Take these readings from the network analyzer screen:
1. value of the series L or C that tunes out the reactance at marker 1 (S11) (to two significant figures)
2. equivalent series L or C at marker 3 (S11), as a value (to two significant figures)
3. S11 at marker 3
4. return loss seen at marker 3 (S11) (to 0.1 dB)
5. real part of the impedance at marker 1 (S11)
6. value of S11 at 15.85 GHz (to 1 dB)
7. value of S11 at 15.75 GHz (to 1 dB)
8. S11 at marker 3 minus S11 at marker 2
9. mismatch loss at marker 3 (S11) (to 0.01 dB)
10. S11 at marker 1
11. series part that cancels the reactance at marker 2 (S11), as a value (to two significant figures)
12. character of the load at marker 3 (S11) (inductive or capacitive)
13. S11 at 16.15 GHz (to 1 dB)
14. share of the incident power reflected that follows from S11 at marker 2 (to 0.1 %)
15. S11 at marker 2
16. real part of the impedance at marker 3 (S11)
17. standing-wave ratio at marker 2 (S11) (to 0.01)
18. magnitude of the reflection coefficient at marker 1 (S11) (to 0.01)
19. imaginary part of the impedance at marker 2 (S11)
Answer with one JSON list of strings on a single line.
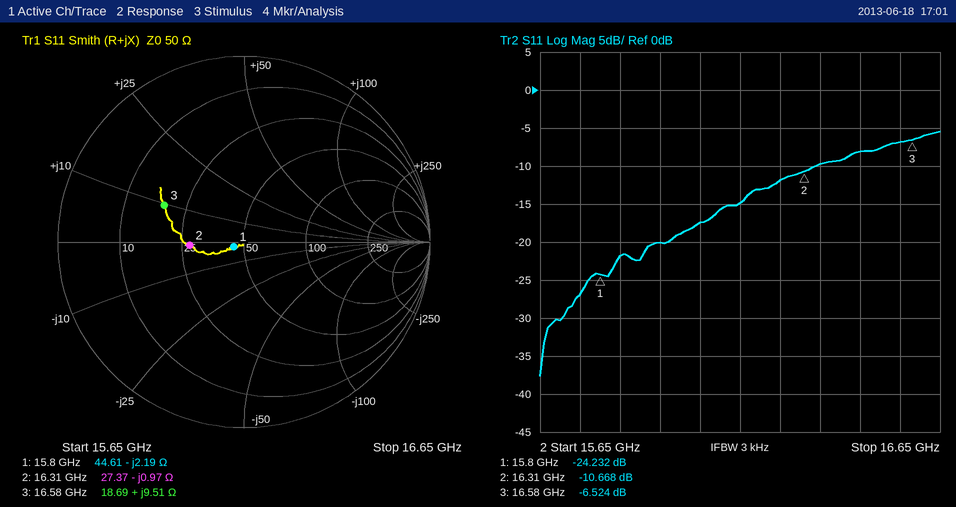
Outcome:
["22 pH", "91 pH", "-6.524 dB", "6.5 dB", "44.61 Ω", "-22 dB", "-27 dB", "4.144 dB", "1.09 dB", "-24.232 dB", "9.5 pH", "inductive", "-15 dB", "8.6 %", "-10.668 dB", "18.69 Ω", "1.83", "0.06", "-0.97 Ω"]
